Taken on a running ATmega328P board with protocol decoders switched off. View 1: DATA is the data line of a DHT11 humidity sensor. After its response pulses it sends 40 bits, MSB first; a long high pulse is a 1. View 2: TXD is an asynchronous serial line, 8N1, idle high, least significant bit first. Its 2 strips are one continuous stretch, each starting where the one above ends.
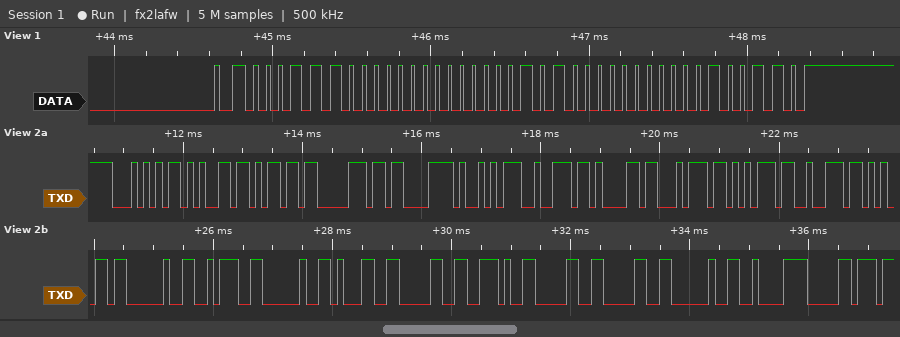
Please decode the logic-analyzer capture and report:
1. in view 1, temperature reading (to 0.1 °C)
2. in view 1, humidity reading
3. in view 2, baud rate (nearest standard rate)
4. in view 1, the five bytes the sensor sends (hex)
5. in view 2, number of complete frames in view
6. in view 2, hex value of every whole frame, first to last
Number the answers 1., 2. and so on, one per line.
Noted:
1. 10.0 °C
2. 28 %
3. 9600 baud
4. 1C 00 0A 00 26
5. 23
6. 54 65 6D 70 C3 A9 72 61 74 75 72 65 20 3A 20 31 30 2E 30 30 20 C2 B0
